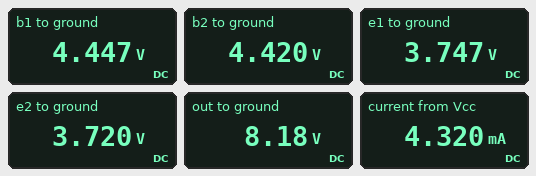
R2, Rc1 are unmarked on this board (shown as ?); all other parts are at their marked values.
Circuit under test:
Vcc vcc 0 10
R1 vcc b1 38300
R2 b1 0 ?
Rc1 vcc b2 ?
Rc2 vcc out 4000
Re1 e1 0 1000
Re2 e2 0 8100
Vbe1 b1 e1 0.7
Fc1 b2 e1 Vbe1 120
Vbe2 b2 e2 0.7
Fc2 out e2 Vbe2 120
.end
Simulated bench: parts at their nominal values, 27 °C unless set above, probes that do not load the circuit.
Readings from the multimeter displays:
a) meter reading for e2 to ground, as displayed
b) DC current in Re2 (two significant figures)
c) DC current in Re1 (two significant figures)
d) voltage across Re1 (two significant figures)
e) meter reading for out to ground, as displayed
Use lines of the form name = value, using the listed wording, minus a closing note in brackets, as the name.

meter reading for e2 to ground, as displayed = 3.720 V
DC current in Re2 = 460 µA
DC current in Re1 = 3.7 mA
voltage across Re1 = 3.7 V
meter reading for out to ground, as displayed = 8.18 V
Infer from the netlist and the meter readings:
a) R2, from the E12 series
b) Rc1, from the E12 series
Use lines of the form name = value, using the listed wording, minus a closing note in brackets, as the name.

R2, from the E12 series = 39 kΩ
Rc1, from the E12 series = 1.5 kΩ
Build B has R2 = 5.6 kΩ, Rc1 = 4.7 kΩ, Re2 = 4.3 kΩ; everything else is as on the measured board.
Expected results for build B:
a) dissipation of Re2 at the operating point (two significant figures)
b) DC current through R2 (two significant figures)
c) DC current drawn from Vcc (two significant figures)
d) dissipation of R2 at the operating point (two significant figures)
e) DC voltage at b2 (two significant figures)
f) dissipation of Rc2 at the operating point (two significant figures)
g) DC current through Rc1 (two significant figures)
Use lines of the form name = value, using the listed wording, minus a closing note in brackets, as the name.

dissipation of Re2 at the operating point = 10 mW
DC current through R2 = 220 µA
DC current drawn from Vcc = 2.3 mA
dissipation of R2 at the operating point = 280 µW
DC voltage at b2 = 7.4 V
dissipation of Rc2 at the operating point = 9.4 mW
DC current through Rc1 = 560 µA
